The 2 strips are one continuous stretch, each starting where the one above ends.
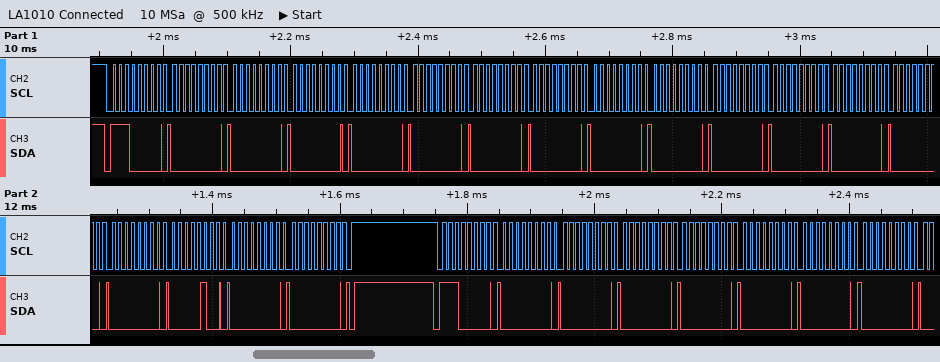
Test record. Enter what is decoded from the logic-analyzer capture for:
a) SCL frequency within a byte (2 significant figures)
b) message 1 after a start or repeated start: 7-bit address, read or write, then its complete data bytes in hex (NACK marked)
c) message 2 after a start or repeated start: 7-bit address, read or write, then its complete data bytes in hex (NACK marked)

100 kHz
0x70 write: 00 00 00 00 00 00 00 00 00 00 00 00 00 00 04 00 00
0x70 write: 00 00 00 00 00 00 00
